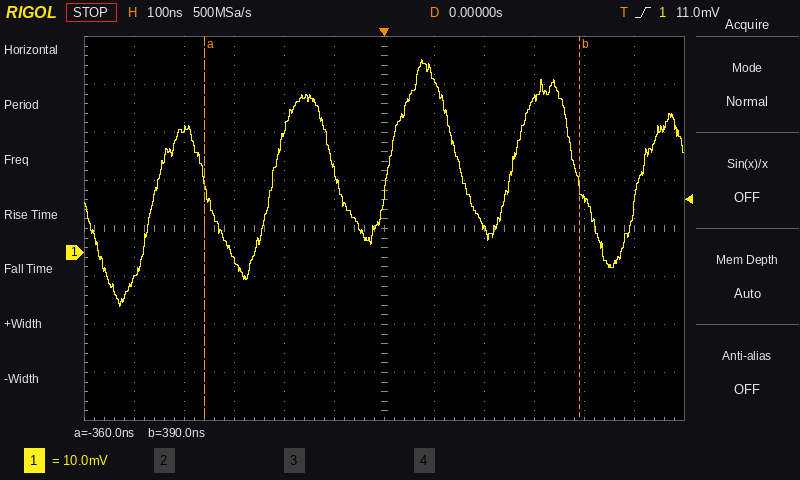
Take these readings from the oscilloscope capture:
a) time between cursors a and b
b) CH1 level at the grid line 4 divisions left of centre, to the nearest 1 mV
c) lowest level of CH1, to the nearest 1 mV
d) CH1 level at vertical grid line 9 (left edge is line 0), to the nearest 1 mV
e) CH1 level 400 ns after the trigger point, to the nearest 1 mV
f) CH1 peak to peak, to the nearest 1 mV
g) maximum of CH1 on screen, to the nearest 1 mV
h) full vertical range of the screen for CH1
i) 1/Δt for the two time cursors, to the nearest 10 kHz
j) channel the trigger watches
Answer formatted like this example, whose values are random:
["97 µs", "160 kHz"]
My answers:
["750 ns", "26 mV", "-11 mV", "32 mV", "11 mV", "51 mV", "40 mV", "80 mV", "1.33 MHz", "CH1"]
